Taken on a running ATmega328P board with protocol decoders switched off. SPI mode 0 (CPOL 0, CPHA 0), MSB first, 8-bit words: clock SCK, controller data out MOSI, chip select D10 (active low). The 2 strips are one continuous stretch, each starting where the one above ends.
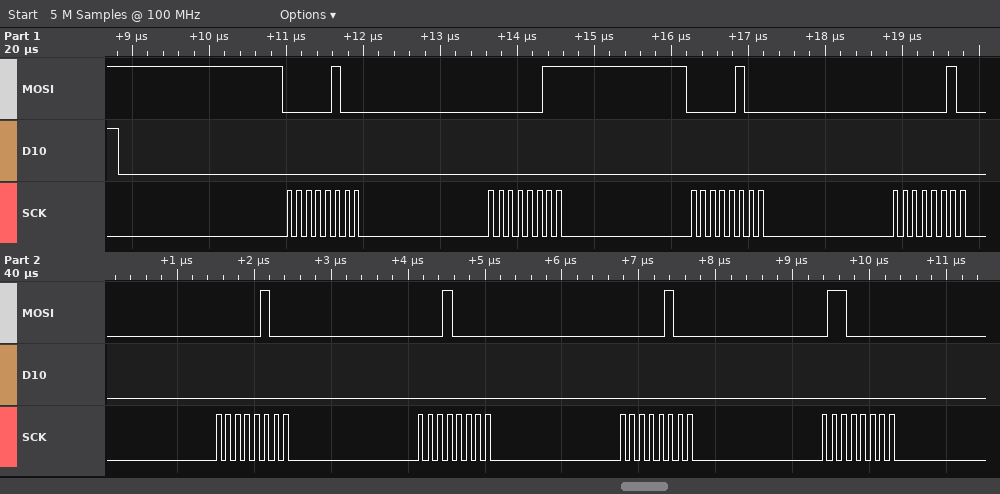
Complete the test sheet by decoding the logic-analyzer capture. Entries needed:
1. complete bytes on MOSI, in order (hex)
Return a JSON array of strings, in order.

["0x04 0x03 0x04 0x02 0x04 0x10 0x04 0x60"]
